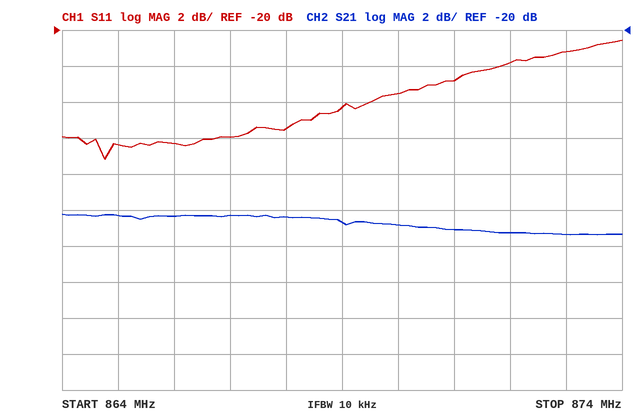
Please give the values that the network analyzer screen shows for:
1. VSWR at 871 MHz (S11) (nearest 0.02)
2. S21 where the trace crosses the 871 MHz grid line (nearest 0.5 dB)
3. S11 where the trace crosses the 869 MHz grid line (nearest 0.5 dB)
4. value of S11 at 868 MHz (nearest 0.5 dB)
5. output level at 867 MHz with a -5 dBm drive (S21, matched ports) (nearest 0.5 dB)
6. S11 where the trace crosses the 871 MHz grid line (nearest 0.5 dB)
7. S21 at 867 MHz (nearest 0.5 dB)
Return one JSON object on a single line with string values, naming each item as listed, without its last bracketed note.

{"VSWR at 871 MHz (S11)": "1.16", "S21 where the trace crosses the 871 MHz grid line": "-31.0 dB", "S11 where the trace crosses the 869 MHz grid line": "-24.5 dB", "value of S11 at 868 MHz": "-25.5 dB", "output level at 867 MHz with a -5 dBm drive (S21, matched ports)": "-35.5 dBm", "S11 where the trace crosses the 871 MHz grid line": "-23.0 dB", "S21 at 867 MHz": "-30.5 dB"}
